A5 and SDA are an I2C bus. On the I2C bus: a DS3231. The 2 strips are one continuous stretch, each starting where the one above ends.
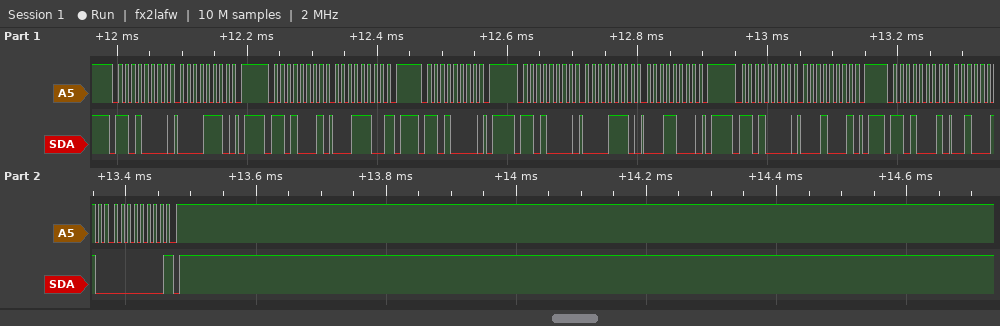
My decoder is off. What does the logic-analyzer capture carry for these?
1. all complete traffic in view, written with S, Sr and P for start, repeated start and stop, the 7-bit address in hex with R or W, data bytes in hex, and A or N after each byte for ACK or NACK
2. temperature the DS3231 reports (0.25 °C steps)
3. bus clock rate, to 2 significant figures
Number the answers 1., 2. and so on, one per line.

1. S 68W A 0E A P S 68R A 1C N P S 68W A P S 68W A 0E A 18 A P S 68W A 11 A P S 68R A 22 A 00 N P
2. 34.00 °C
3. 100 kHz
